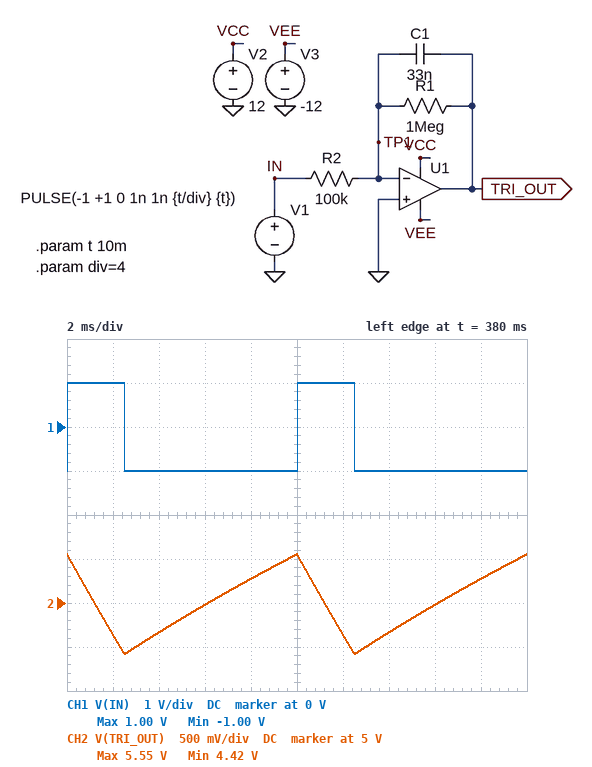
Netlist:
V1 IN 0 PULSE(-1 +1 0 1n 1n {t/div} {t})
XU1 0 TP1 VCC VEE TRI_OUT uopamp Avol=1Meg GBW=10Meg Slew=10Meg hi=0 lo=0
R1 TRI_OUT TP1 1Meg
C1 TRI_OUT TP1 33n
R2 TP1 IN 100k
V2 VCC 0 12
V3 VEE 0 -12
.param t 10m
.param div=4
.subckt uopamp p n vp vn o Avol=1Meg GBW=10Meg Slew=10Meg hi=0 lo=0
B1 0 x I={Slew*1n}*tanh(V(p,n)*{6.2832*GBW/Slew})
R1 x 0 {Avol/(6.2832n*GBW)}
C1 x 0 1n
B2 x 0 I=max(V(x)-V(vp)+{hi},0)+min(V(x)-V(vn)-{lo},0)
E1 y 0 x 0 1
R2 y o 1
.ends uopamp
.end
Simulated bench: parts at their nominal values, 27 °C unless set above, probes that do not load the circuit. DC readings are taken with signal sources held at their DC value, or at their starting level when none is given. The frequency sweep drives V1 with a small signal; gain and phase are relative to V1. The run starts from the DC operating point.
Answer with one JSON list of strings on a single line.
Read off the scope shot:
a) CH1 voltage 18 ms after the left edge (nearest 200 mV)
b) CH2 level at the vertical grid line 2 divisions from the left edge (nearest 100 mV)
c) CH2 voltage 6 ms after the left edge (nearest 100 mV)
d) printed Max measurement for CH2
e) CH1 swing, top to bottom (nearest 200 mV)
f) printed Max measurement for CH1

["-1.0 V", "4.7 V", "5.0 V", "5.55 V", "2.0 V", "1.00 V"]
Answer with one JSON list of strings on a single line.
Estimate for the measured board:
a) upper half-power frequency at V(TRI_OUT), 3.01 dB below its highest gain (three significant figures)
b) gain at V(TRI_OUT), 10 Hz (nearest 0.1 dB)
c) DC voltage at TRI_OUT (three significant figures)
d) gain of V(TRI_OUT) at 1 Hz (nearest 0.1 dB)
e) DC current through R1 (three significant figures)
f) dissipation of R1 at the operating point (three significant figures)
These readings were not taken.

["4.82 Hz", "12.8 dB", "10.0 V", "19.8 dB", "10.0 µA", "100 µW"]
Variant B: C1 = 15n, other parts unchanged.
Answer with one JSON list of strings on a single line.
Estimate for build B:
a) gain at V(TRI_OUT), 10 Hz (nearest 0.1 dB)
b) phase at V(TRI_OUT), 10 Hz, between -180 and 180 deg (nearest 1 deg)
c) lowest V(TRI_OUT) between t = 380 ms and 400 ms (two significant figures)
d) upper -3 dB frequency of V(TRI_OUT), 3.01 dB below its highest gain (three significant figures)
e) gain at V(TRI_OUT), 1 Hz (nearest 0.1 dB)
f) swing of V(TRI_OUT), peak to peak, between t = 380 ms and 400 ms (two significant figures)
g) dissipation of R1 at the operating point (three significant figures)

["17.2 dB", "137 deg", "3.7 V", "10.6 Hz", "20.0 dB", "2.5 V", "100 µW"]
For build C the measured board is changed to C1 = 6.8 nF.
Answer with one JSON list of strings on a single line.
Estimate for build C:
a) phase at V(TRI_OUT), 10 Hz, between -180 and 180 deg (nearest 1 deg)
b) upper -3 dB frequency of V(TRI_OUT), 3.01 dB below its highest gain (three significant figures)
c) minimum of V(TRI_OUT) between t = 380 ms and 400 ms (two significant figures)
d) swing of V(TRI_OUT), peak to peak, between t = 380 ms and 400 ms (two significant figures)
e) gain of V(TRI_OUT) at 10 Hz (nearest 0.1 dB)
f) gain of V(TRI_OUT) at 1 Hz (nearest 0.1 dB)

["157 deg", "23.4 Hz", "2.0 V", "5.3 V", "19.3 dB", "20.0 dB"]
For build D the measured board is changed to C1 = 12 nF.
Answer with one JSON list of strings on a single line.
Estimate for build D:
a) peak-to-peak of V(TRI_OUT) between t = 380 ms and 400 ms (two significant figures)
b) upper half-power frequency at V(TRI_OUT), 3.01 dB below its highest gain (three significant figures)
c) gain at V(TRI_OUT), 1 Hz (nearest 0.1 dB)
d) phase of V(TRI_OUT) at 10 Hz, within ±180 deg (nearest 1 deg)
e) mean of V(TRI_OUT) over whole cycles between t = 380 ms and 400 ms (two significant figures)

["3.1 V", "13.3 Hz", "20.0 dB", "143 deg", "5.0 V"]
